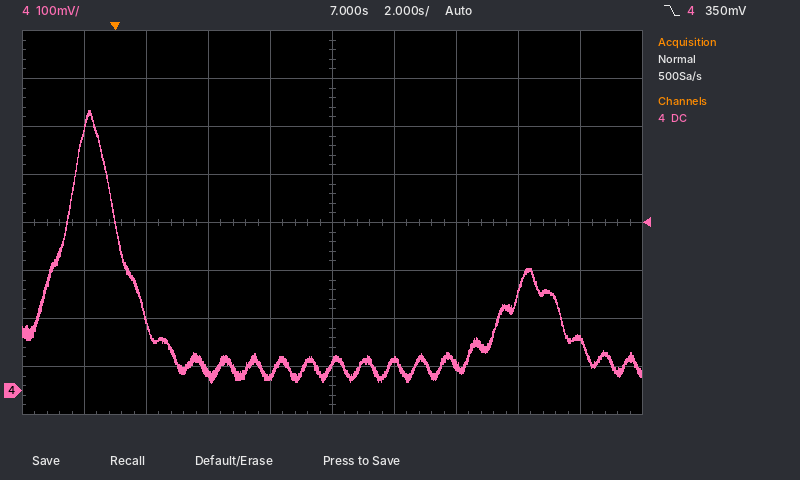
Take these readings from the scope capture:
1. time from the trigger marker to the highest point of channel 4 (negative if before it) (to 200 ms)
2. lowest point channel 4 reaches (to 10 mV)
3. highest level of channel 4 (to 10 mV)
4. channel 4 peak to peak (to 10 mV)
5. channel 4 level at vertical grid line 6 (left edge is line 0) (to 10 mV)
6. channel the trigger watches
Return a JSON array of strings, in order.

["-800 ms", "10 mV", "580 mV", "570 mV", "60 mV", "channel 4"]
